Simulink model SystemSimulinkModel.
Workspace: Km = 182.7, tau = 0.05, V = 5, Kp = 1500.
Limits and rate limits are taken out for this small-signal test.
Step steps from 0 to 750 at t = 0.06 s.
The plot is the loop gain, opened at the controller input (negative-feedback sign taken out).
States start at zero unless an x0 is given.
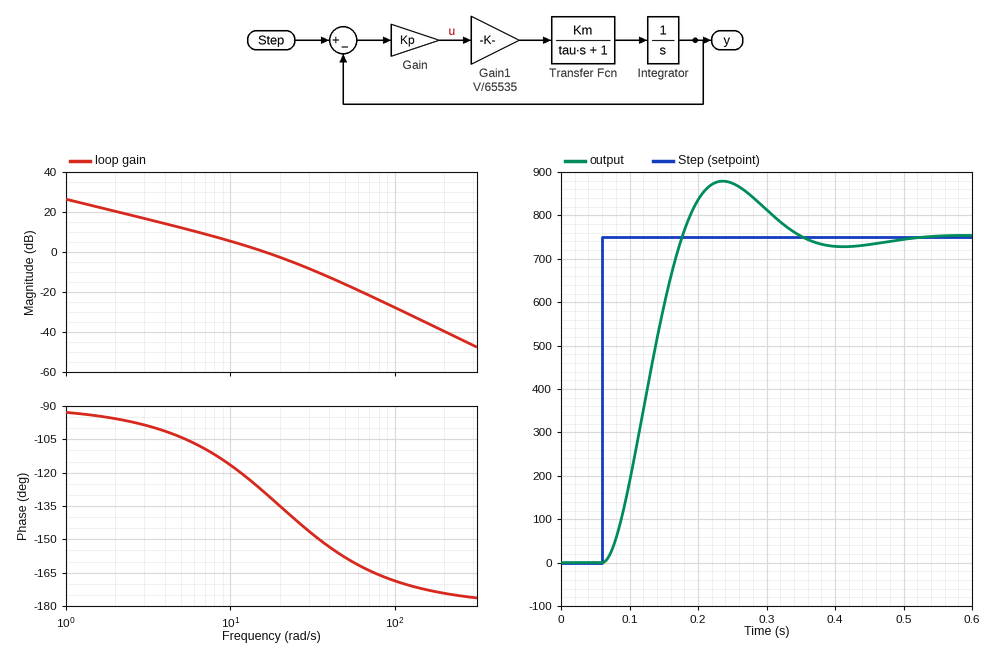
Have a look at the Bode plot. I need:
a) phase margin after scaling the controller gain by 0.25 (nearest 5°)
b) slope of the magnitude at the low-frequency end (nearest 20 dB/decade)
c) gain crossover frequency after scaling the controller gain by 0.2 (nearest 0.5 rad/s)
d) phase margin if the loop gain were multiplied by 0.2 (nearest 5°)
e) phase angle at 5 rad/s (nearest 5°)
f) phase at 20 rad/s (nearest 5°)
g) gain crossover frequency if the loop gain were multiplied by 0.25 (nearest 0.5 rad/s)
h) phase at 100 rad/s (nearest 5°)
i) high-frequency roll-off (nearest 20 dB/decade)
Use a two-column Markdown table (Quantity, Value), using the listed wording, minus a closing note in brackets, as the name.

| Quantity | Value |
|---|---|
| phase margin after scaling the controller gain by 0.25 | 75° |
| slope of the magnitude at the low-frequency end | -20 dB/decade |
| gain crossover frequency after scaling the controller gain by 0.2 | 4.0 rad/s |
| phase margin if the loop gain were multiplied by 0.2 | 80° |
| phase angle at 5 rad/s | -105° |
| phase at 20 rad/s | -135° |
| gain crossover frequency if the loop gain were multiplied by 0.25 | 5.0 rad/s |
| phase at 100 rad/s | -170° |
| high-frequency roll-off | -40 dB/decade |
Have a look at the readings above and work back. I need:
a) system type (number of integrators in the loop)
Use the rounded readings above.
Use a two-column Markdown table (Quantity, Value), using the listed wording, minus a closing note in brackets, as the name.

| Quantity | Value |
|---|---|
| system type | 1 |
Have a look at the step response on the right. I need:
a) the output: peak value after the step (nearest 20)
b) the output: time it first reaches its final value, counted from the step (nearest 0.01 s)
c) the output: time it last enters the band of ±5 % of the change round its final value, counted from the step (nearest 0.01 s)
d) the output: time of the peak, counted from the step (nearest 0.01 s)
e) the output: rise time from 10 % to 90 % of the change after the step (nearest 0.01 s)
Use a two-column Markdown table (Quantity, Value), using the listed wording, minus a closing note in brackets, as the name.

| Quantity | Value |
|---|---|
| the output: peak value after the step | 880 |
| the output: time it first reaches its final value, counted from the step | 0.12 s |
| the output: time it last enters the band of ±5 % of the change round its final value, counted from the step | 0.26 s |
| the output: time of the peak, counted from the step | 0.18 s |
| the output: rise time from 10 % to 90 % of the change after the step | 0.08 s |
